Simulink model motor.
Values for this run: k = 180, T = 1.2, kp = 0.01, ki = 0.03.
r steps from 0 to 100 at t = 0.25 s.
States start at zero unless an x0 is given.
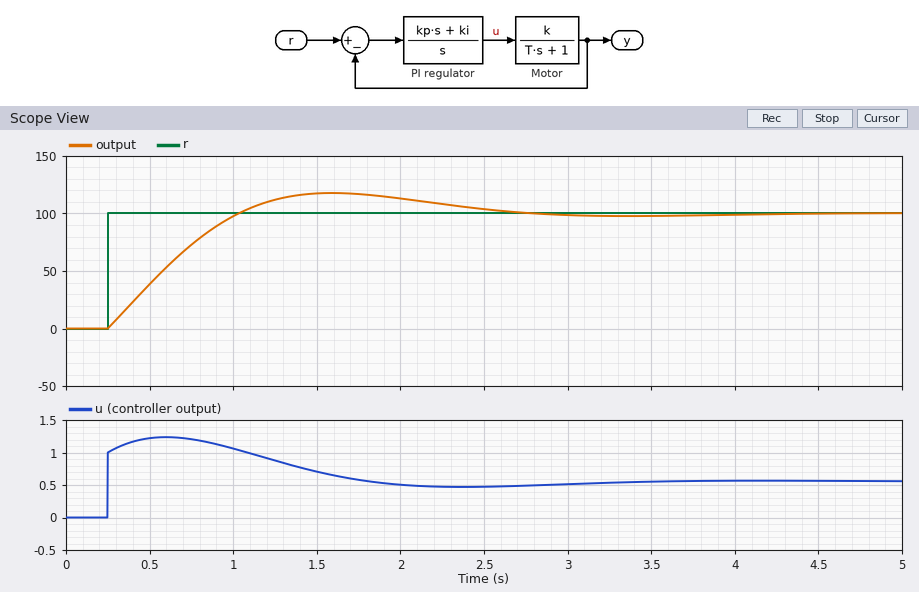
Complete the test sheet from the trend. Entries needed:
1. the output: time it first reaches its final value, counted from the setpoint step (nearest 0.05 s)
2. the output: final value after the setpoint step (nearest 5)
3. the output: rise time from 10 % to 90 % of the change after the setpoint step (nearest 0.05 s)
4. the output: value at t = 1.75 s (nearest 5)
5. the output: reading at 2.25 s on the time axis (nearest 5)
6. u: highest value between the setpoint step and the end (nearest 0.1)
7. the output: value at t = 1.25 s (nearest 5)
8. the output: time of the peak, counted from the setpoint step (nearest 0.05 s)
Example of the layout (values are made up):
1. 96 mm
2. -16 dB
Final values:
1. 0.80 s
2. 100
3. 0.60 s
4. 115
5. 110
6. 1.2
7. 110
8. 1.35 s
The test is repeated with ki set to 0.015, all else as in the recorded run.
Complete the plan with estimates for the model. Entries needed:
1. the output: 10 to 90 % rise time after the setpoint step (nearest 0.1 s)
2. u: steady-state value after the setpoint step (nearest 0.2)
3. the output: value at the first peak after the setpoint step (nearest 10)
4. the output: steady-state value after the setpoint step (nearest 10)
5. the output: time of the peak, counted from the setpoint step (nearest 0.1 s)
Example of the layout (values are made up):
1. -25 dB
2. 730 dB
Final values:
1. 0.9 s
2. 0.6
3. 110
4. 100
5. 2.0 s
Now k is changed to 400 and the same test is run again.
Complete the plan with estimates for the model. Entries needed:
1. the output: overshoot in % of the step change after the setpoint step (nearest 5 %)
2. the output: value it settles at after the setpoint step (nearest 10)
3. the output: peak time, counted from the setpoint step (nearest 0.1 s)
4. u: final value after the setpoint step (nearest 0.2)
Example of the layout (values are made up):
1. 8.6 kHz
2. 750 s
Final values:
1. 15 %
2. 100
3. 0.8 s
4. 0.2
